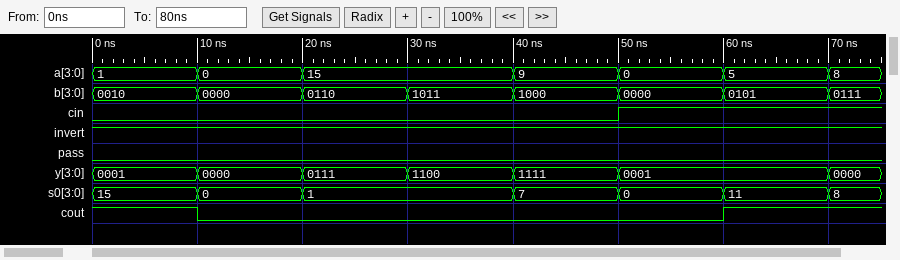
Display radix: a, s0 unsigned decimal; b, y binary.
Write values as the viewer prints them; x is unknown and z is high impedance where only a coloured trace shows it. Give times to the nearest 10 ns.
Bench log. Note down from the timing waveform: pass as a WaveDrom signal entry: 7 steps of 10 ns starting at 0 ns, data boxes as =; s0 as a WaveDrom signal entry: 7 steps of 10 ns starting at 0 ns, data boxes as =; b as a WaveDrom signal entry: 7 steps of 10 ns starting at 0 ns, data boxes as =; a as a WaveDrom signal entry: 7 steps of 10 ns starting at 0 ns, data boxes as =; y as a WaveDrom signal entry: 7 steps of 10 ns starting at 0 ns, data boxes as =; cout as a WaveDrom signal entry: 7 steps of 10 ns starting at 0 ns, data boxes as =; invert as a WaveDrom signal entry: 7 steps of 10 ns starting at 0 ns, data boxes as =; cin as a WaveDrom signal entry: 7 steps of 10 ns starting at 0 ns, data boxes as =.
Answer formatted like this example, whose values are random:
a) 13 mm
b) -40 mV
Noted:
a) {name: 'pass', wave: '0......'}
b) {name: 's0', wave: '===.===', data: '15 0 1 7 0 11'}
c) {name: 'b', wave: '=======', data: '0010 0000 0110 1011 1000 0000 0101'}
d) {name: 'a', wave: '===.===', data: '1 0 15 9 0 5'}
e) {name: 'y', wave: '======.', data: '0001 0000 0111 1100 1111 0001'}
f) {name: 'cout', wave: '10....1'}
g) {name: 'invert', wave: '1......'}
h) {name: 'cin', wave: '0....1.'}
